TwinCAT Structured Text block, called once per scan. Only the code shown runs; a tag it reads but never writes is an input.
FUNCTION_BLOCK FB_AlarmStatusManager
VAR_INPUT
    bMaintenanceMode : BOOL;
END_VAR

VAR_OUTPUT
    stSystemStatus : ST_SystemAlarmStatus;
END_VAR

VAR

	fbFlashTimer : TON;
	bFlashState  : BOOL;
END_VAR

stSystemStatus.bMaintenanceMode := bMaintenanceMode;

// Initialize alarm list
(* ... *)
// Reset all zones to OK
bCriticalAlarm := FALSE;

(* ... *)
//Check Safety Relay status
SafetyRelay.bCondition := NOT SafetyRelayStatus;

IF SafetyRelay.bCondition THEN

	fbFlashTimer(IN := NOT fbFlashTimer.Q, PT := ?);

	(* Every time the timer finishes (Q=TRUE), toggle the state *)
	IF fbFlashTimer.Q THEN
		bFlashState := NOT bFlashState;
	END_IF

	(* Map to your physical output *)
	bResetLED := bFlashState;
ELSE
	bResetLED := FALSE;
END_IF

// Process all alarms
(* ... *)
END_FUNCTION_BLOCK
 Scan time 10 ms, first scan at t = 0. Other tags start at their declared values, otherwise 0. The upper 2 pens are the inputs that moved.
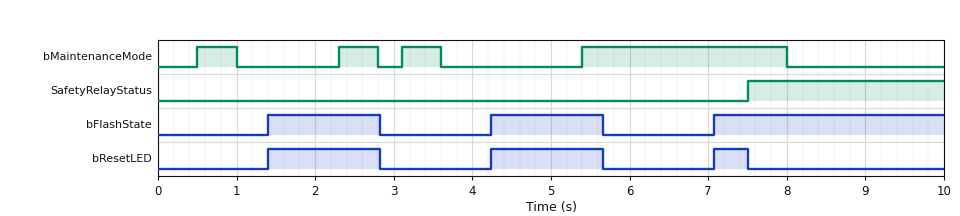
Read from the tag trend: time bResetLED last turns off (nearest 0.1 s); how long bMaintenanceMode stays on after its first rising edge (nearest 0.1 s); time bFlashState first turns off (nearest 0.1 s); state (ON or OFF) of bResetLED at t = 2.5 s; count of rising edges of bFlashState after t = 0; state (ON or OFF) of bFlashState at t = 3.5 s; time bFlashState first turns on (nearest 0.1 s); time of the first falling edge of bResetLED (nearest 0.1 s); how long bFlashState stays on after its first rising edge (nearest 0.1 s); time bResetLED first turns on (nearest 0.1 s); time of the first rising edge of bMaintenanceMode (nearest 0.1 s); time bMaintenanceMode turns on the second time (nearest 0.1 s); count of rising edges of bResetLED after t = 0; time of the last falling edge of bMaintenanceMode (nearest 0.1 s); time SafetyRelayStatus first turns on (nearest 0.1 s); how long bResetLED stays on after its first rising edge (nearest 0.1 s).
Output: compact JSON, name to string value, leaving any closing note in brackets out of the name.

{"time bResetLED last turns off": "7.5 s", "how long bMaintenanceMode stays on after its first rising edge": "0.5 s", "time bFlashState first turns off": "2.8 s", "state (ON or OFF) of bResetLED at t = 2.5 s": "ON", "count of rising edges of bFlashState after t = 0": "3", "state (ON or OFF) of bFlashState at t = 3.5 s": "OFF", "time bFlashState first turns on": "1.4 s", "time of the first falling edge of bResetLED": "2.8 s", "how long bFlashState stays on after its first rising edge": "1.4 s", "time bResetLED first turns on": "1.4 s", "time of the first rising edge of bMaintenanceMode": "0.5 s", "time bMaintenanceMode turns on the second time": "2.3 s", "count of rising edges of bResetLED after t = 0": "3", "time of the last falling edge of bMaintenanceMode": "8.0 s", "time SafetyRelayStatus first turns on": "7.5 s", "how long bResetLED stays on after its first rising edge": "1.4 s"}
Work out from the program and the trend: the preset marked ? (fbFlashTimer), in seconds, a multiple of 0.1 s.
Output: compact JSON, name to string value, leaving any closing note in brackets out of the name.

{"the preset marked ? (fbFlashTimer), in seconds, a multiple of 0.1 s": "1.4 s"}
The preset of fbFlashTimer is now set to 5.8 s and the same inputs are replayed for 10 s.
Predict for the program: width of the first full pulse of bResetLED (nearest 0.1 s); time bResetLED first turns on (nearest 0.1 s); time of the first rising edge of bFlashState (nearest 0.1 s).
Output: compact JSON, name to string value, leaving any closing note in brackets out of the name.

{"width of the first full pulse of bResetLED": "1.7 s", "time bResetLED first turns on": "5.8 s", "time of the first rising edge of bFlashState": "5.8 s"}
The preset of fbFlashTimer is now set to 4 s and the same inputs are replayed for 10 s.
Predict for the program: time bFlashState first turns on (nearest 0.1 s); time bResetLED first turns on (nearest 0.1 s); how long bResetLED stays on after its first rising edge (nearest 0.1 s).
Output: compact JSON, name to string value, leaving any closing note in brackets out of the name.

{"time bFlashState first turns on": "4.0 s", "time bResetLED first turns on": "4.0 s", "how long bResetLED stays on after its first rising edge": "3.5 s"}
